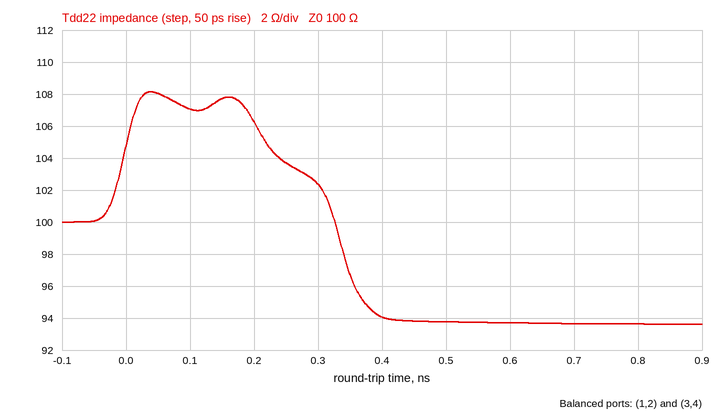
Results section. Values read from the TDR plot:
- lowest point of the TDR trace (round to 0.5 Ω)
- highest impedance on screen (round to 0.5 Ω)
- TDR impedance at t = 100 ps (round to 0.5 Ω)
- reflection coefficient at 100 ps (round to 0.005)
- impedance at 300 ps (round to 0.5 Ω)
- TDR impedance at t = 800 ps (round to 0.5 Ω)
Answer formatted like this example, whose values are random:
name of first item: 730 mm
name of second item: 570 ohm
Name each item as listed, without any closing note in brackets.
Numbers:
lowest point of the TDR trace: 93.5 Ω
highest impedance on screen: 108.0 Ω
TDR impedance at t = 100 ps: 107.0 Ω
reflection coefficient at 100 ps: +0.035
impedance at 300 ps: 102.5 Ω
TDR impedance at t = 800 ps: 93.5 Ω
